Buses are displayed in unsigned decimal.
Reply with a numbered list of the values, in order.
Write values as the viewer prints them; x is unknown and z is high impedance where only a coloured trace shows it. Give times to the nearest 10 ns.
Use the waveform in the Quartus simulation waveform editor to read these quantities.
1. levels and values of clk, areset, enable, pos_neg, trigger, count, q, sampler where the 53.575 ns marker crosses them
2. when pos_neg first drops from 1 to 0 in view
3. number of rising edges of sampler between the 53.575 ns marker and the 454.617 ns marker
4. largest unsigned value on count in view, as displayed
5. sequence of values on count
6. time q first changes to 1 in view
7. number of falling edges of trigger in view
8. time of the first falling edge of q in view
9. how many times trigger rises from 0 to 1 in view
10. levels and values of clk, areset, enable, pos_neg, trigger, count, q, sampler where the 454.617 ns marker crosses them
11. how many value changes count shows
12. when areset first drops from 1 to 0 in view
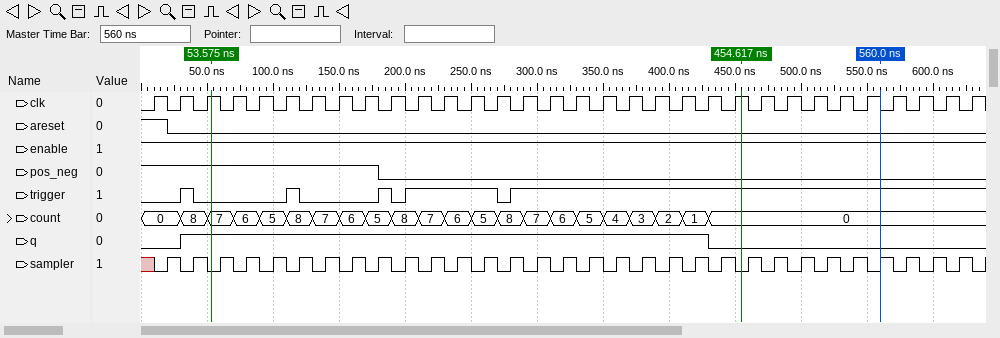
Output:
1. clk=1, areset=0, enable=1, pos_neg=1, trigger=0, count=7, q=1, sampler=0
2. 180 ns
3. 20
4. 8
5. 0, 8, 7, 6, 5, 8, 7, 6, 5, 8, 7, 6, 5, 8, 7, 6, 5, 4, 3, 2, 1, 0
6. 30 ns
7. 4
8. 430 ns
9. 5
10. clk=1, areset=0, enable=1, pos_neg=0, trigger=1, count=0, q=0, sampler=0
11. 21
12. 20 ns
